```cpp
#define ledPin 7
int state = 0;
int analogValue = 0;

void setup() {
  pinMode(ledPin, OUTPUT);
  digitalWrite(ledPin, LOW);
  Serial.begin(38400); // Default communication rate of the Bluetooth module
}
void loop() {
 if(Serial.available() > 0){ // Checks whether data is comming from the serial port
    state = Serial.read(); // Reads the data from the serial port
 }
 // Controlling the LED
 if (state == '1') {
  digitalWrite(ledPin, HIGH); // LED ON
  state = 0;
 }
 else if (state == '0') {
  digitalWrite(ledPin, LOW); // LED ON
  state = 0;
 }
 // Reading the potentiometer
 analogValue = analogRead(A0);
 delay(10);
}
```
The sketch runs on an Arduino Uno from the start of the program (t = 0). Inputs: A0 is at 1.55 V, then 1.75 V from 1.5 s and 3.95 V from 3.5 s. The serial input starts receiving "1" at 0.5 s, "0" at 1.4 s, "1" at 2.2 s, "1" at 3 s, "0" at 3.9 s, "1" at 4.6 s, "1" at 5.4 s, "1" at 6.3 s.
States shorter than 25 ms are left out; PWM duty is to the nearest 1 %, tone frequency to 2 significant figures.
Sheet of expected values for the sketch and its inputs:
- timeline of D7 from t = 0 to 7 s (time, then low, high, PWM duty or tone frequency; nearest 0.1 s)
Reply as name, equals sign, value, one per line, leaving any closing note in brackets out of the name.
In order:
timeline of D7 from t = 0 to 7 s = 0 s low; 0.5 s high; 1.4 s low; 2.2 s high; 3.9 s low; 4.6 s high
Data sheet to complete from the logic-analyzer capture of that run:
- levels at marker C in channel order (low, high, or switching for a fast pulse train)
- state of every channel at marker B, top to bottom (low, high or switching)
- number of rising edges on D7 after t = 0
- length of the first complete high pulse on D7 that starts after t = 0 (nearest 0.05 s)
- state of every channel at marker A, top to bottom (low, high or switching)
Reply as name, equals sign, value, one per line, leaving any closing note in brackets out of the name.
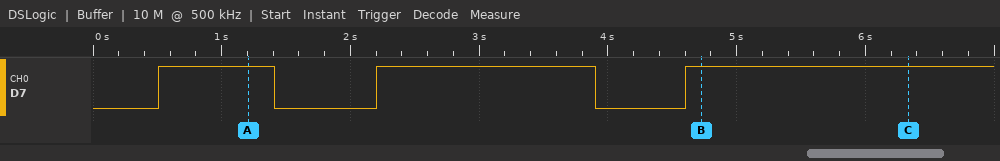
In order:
levels at marker C in channel order = D7 high
state of every channel at marker B, top to bottom = D7 high
number of rising edges on D7 after t = 0 = 3
length of the first complete high pulse on D7 that starts after t = 0 = 0.90 s
state of every channel at marker A, top to bottom = D7 high
